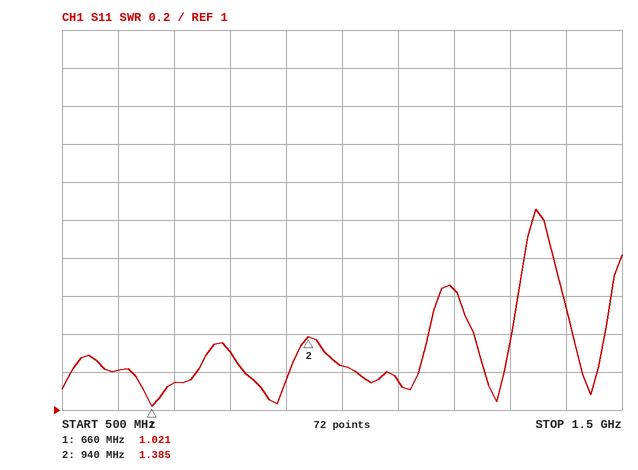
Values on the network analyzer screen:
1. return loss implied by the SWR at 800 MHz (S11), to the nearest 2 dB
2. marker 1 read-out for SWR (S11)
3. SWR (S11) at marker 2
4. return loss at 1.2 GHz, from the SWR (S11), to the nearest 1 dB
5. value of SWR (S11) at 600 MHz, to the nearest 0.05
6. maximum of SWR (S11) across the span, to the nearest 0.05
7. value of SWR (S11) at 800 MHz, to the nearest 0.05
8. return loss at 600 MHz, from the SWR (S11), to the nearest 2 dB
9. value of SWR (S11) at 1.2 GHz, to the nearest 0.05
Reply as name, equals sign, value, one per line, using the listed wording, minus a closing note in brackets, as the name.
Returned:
return loss implied by the SWR at 800 MHz (S11), to the nearest 2 dB = 18 dB
marker 1 read-out for SWR = 1.021
SWR (S11) at marker 2 = 1.385
return loss at 1.2 GHz, from the SWR (S11), to the nearest 1 dB = 12 dB
value of SWR (S11) at 600 MHz, to the nearest 0.05 = 1.20
maximum of SWR (S11) across the span, to the nearest 0.05 = 2.05
value of SWR (S11) at 800 MHz, to the nearest 0.05 = 1.30
return loss at 600 MHz, from the SWR (S11), to the nearest 2 dB = 20 dB
value of SWR (S11) at 1.2 GHz, to the nearest 0.05 = 1.65
